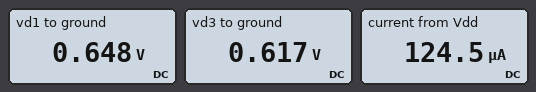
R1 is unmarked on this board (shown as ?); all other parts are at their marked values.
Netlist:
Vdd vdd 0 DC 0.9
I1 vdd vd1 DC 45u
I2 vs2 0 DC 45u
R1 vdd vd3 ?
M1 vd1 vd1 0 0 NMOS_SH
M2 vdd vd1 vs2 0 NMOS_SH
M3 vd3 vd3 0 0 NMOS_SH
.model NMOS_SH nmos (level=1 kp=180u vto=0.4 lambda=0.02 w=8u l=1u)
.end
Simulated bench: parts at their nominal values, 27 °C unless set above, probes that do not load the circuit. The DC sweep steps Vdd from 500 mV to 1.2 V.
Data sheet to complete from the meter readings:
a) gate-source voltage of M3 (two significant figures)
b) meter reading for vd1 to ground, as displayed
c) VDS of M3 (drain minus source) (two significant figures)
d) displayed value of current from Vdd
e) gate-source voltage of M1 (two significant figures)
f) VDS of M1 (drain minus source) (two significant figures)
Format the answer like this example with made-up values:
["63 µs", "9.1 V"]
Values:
["620 mV", "0.648 V", "620 mV", "124.5 µA", "650 mV", "650 mV"]
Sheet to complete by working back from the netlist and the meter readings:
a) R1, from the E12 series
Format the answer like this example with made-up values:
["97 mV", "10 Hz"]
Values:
["8.2 kΩ"]
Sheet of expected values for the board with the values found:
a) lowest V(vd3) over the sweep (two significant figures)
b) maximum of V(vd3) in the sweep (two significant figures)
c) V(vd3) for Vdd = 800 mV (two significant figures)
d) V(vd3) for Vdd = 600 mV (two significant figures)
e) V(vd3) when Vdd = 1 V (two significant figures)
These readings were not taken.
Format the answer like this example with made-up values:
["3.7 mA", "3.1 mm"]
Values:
["470 mV", "690 mV", "590 mV", "520 mV", "640 mV"]
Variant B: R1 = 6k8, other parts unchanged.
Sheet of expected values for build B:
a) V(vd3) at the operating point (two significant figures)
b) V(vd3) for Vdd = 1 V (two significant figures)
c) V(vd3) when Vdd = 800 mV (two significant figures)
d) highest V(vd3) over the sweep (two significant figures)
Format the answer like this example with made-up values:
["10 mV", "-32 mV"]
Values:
["630 mV", "660 mV", "600 mV", "710 mV"]
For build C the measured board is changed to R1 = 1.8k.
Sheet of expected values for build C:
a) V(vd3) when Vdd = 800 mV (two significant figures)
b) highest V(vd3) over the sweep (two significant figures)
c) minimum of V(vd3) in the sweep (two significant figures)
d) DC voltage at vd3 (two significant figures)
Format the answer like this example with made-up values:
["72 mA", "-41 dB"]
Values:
["690 mV", "890 mV", "490 mV", "740 mV"]
